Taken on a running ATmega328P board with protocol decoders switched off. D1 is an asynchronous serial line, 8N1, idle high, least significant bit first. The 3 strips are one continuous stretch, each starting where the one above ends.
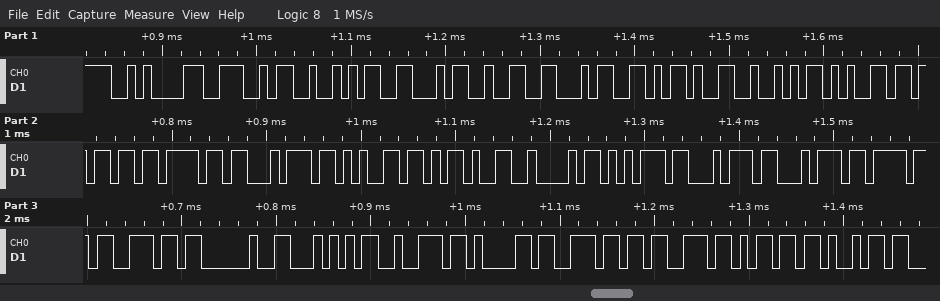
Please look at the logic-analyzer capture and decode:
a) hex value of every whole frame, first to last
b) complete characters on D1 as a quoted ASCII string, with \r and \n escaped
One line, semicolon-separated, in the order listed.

0x0A 0x4E 0x52 0x46 0x32 0x34 0x2D 0x52 0x65 0x6D 0x6F 0x74 0x65 0x2D 0x42 0x75 0x74 0x74 0x6F 0x6E 0x20 0x54 0x72 0x61 0x6E 0x73 0x6D 0x69; "\nNRF24-Remote-Button Transmi"
